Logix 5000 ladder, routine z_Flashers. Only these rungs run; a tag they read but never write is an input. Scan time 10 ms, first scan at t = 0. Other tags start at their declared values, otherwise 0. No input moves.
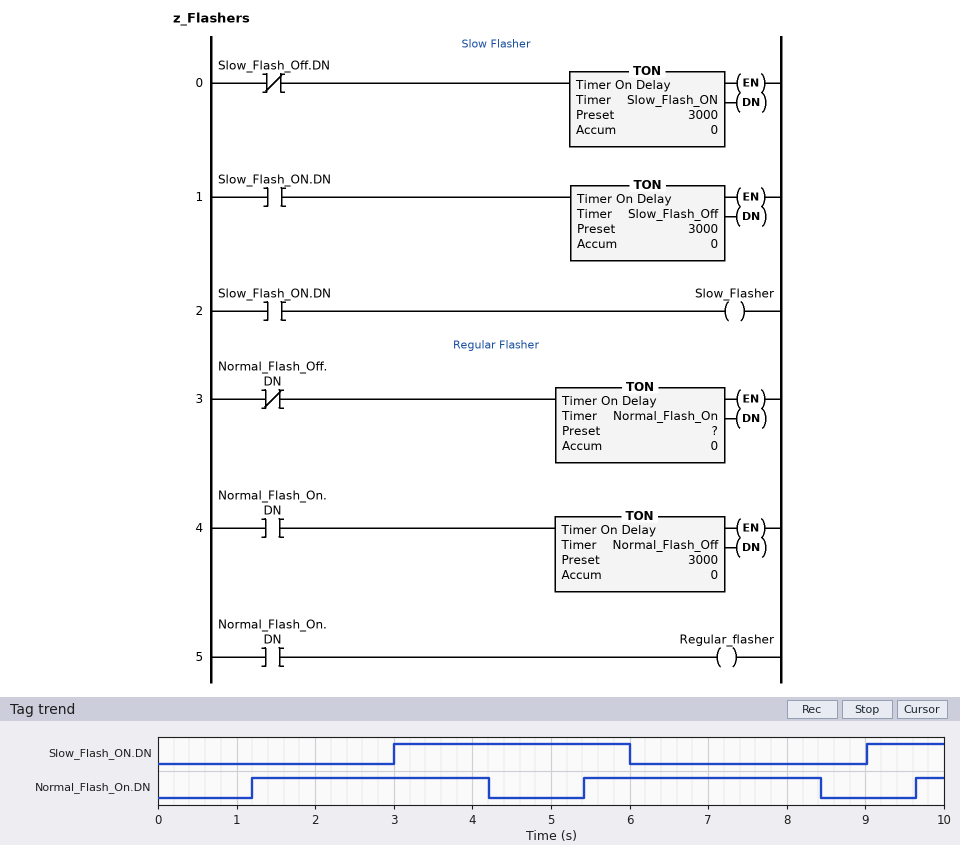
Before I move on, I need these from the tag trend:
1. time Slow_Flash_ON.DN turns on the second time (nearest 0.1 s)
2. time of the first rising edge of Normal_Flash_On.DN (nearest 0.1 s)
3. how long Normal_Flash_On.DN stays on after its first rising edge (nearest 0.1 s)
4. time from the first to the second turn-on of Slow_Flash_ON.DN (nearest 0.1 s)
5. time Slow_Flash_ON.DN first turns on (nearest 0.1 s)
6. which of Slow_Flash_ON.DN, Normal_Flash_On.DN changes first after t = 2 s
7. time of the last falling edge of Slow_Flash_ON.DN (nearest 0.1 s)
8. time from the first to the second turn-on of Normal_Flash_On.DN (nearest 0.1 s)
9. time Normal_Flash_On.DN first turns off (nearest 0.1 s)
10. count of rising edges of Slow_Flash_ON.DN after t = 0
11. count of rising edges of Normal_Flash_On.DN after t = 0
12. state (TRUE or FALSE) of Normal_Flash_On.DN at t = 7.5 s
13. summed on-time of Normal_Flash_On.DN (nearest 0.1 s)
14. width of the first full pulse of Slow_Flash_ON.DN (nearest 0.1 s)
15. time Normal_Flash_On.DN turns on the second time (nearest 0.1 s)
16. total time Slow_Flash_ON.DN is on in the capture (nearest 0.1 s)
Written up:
9.0 s
1.2 s
3.0 s
6.0 s
3.0 s
Slow_Flash_ON.DN
6.0 s
4.2 s
4.2 s
2
3
TRUE
6.4 s
3.0 s
5.4 s
4.0 s
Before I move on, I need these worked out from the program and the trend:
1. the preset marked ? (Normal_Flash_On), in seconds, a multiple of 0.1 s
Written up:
1.2 s
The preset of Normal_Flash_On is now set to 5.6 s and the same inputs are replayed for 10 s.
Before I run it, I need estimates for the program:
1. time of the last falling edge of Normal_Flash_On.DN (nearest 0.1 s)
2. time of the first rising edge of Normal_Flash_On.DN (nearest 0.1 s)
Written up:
8.6 s
5.6 s
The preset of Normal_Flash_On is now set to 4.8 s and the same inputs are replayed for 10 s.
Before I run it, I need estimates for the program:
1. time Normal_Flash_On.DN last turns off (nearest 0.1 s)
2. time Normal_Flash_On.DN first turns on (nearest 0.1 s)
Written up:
7.8 s
4.8 s
